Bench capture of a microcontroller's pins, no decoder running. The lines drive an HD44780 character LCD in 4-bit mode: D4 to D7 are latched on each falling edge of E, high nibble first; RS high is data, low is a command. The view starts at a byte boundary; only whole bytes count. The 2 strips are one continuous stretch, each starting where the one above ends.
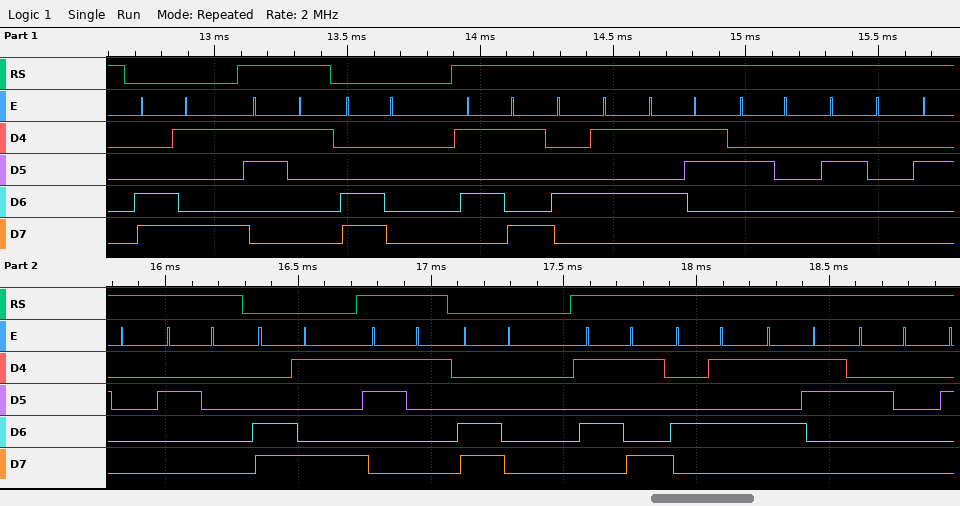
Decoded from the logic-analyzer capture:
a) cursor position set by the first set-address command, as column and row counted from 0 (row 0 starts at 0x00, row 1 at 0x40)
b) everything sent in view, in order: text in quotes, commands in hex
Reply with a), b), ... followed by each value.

a) column 9, row 1
b) 0xC9 "1" 0xC0 "YES    " 0xC9 "1" 0xC0 "YES "
